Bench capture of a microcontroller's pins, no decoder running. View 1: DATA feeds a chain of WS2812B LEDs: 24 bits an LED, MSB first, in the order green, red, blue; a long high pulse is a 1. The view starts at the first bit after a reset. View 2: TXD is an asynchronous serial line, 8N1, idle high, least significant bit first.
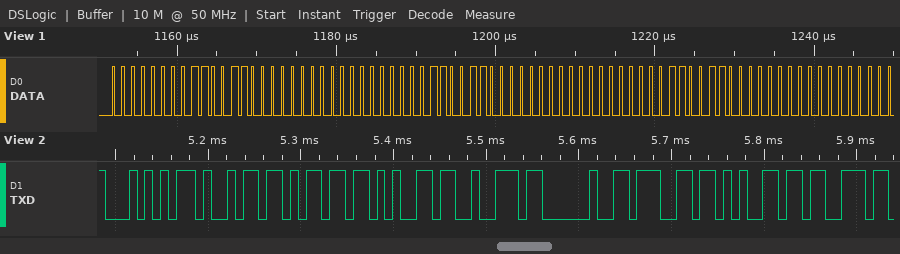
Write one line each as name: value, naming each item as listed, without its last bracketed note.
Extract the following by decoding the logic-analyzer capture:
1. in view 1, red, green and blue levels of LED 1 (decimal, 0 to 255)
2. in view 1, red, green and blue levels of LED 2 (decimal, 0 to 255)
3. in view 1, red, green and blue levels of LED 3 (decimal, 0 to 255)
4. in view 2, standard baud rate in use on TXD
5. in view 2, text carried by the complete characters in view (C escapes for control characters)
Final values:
in view 1, red, green and blue levels of LED 1: 204, 0, 0
in view 1, red, green and blue levels of LED 2: 204, 0, 0
in view 1, red, green and blue levels of LED 3: 204, 0, 0
in view 2, standard baud rate in use on TXD: 115200 baud
in view 2, text carried by the complete characters in view: "Timer ges"
